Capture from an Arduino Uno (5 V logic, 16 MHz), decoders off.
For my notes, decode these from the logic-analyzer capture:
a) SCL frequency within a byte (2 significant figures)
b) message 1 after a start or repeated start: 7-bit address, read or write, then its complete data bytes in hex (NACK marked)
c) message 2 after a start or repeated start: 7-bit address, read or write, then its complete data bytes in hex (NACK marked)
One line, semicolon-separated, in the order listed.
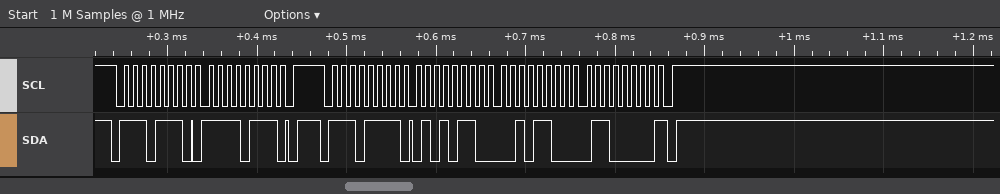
100 kHz; 0x77 write: F7; 0x77 read: 56 2C 60 NACK
